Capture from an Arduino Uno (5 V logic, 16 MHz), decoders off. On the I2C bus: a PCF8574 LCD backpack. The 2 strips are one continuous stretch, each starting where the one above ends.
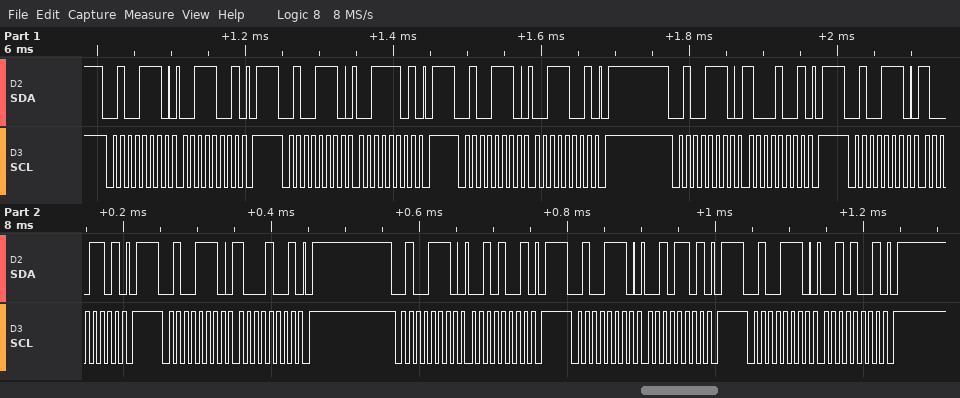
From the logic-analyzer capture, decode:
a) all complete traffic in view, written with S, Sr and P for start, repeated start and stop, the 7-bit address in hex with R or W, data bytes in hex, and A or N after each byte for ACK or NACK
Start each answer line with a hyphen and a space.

- S 27W A 39 A P S 27W A 3D A P S 27W A 39 A P S 27W A 89 A P S 27W A 8D A P S 27W A 89 A P S 27W A 29 A P S 27W A 2D A P S 27W A 29 A P
